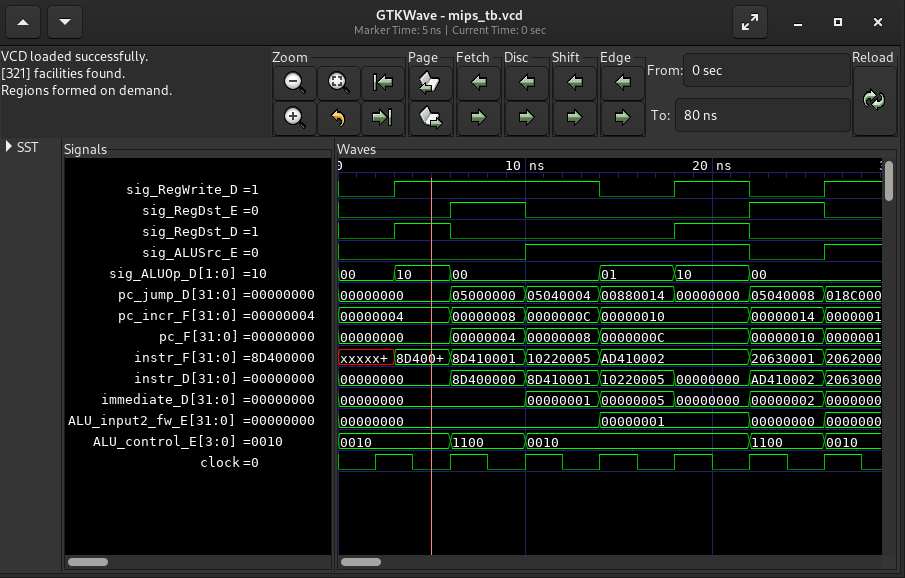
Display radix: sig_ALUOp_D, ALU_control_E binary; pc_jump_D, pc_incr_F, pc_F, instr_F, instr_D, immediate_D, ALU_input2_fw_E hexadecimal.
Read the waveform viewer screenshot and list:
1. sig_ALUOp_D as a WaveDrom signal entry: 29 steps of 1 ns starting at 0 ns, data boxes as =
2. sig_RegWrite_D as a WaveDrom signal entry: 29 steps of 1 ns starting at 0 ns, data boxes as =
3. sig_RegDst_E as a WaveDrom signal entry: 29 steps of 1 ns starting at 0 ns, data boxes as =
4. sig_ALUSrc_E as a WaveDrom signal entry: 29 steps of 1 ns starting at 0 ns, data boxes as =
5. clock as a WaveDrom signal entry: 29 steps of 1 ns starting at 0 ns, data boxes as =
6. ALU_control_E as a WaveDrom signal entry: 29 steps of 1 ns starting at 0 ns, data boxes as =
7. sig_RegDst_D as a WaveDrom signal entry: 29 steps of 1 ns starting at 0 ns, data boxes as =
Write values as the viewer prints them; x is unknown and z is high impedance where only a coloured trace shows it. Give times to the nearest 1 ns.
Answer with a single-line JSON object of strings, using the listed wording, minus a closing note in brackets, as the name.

{"sig_ALUOp_D as a WaveDrom signal entry: 29 steps of 1 ns starting at 0 ns, data boxes as =": "{name: 'sig_ALUOp_D', wave: '=..=..=.......=...=...=......', data: '00 10 00 01 10 00'}", "sig_RegWrite_D as a WaveDrom signal entry: 29 steps of 1 ns starting at 0 ns, data boxes as =": "{name: 'sig_RegWrite_D', wave: '0..1..........0...1...0...1..'}", "sig_RegDst_E as a WaveDrom signal entry: 29 steps of 1 ns starting at 0 ns, data boxes as =": "{name: 'sig_RegDst_E', wave: '0.....1...0...........1...0..'}", "sig_ALUSrc_E as a WaveDrom signal entry: 29 steps of 1 ns starting at 0 ns, data boxes as =": "{name: 'sig_ALUSrc_E', wave: '0.........1...........0...1..'}", "clock as a WaveDrom signal entry: 29 steps of 1 ns starting at 0 ns, data boxes as =": "{name: 'clock', wave: '0.1.0.1.0.1.0.1.0.1.0.1.0.1.0'}", "ALU_control_E as a WaveDrom signal entry: 29 steps of 1 ns starting at 0 ns, data boxes as =": "{name: 'ALU_control_E', wave: '=.....=...=...........=...=..', data: '0010 1100 0010 1100 0010'}", "sig_RegDst_D as a WaveDrom signal entry: 29 steps of 1 ns starting at 0 ns, data boxes as =": "{name: 'sig_RegDst_D', wave: '0..1..0...........1...0......'}"}
